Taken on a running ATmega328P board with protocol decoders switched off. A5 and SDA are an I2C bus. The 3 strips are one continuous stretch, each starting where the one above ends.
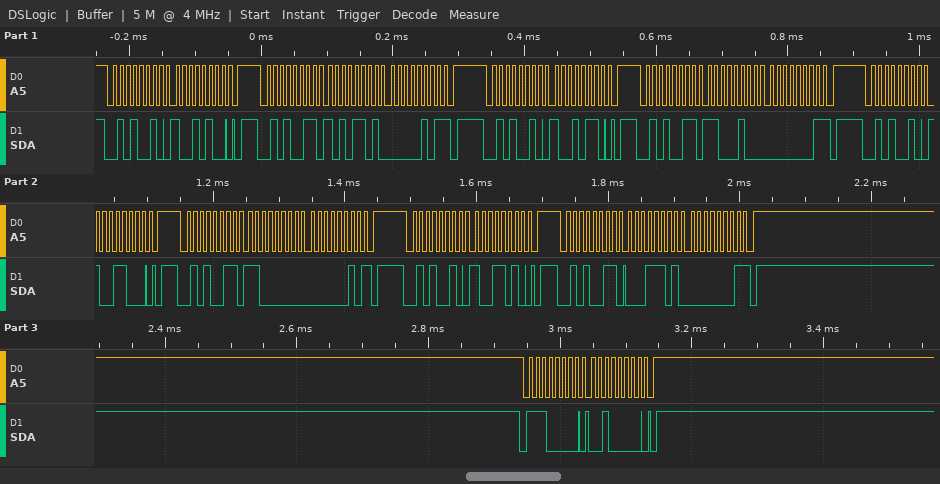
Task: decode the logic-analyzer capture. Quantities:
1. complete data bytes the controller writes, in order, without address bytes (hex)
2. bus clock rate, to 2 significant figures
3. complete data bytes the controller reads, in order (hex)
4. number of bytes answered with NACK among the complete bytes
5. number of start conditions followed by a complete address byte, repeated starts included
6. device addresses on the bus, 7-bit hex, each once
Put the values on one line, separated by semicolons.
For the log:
94 96 98 9A 20; 100 kHz; AD 05 C4 01 C0 02 1D 01; 4; 9; 0x29 0x70
